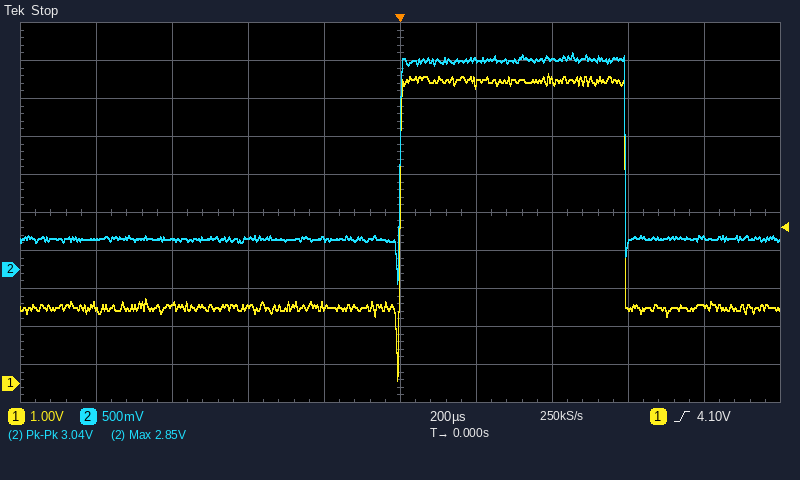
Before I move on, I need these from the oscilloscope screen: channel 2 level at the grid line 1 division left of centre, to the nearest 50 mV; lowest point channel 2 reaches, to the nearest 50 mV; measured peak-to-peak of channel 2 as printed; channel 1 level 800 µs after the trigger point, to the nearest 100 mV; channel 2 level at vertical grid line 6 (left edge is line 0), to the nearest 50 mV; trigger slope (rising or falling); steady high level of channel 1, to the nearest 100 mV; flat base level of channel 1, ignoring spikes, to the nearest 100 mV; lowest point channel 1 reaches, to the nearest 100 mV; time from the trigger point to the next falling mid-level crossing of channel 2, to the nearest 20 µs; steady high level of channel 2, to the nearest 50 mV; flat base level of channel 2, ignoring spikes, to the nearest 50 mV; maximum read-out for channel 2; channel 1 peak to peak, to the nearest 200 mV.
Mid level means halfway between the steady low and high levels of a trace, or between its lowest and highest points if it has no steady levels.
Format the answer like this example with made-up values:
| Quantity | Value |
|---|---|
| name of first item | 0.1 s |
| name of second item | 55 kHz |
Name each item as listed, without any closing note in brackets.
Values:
| Quantity | Value |
|---|---|
| channel 2 level at the grid line 1 division left of centre, to the nearest 50 mV | 400 mV |
| lowest point channel 2 reaches, to the nearest 50 mV | -200 mV |
| measured peak-to-peak of channel 2 as printed | 3.04 V |
| channel 1 level 800 µs after the trigger point, to the nearest 100 mV | 2.0 V |
| channel 2 level at vertical grid line 6 (left edge is line 0), to the nearest 50 mV | 2.75 V |
| trigger slope | rising |
| steady high level of channel 1, to the nearest 100 mV | 8.0 V |
| flat base level of channel 1, ignoring spikes, to the nearest 100 mV | 2.0 V |
| lowest point channel 1 reaches, to the nearest 100 mV | 100 mV |
| time from the trigger point to the next falling mid-level crossing of channel 2, to the nearest 20 µs | 600 µs |
| steady high level of channel 2, to the nearest 50 mV | 2.75 V |
| flat base level of channel 2, ignoring spikes, to the nearest 50 mV | 400 mV |
| maximum read-out for channel 2 | 2.85 V |
| channel 1 peak to peak, to the nearest 200 mV | 8.0 V |
